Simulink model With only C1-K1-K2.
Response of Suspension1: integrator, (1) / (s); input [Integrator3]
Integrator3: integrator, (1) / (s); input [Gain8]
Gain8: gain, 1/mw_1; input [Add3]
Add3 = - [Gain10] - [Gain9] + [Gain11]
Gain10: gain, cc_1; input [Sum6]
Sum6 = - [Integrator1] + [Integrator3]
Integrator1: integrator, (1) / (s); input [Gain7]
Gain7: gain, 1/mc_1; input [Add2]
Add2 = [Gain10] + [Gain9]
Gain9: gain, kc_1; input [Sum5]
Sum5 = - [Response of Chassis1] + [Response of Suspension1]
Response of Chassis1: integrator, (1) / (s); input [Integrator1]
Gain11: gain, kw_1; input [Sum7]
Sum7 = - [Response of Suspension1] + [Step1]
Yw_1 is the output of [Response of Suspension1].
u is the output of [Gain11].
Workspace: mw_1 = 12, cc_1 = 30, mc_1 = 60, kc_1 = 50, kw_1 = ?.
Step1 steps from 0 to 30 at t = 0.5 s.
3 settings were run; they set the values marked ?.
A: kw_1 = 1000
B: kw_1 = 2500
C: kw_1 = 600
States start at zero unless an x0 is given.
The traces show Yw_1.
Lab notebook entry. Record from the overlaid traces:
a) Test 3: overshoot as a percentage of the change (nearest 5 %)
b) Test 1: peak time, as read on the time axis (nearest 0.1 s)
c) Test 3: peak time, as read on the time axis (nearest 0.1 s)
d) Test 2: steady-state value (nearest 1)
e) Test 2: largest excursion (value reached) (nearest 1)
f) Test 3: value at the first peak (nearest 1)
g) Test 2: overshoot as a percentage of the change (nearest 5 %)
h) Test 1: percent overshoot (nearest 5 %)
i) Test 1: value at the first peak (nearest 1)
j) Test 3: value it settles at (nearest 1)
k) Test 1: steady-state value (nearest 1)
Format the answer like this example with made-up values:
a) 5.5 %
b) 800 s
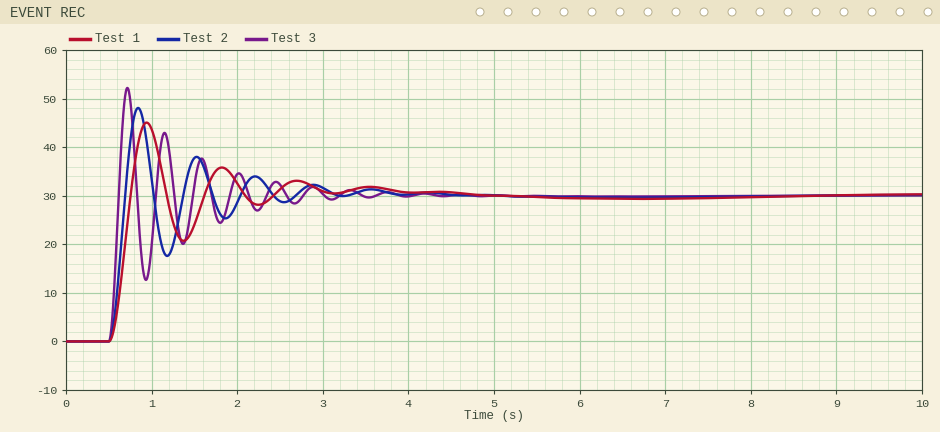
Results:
a) 75 %
b) 0.9 s
c) 0.7 s
d) 30
e) 48
f) 52
g) 60 %
h) 50 %
i) 45
j) 30
k) 30
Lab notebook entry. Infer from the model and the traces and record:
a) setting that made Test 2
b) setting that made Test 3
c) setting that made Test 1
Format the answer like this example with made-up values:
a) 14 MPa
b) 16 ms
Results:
a) A
b) B
c) C
